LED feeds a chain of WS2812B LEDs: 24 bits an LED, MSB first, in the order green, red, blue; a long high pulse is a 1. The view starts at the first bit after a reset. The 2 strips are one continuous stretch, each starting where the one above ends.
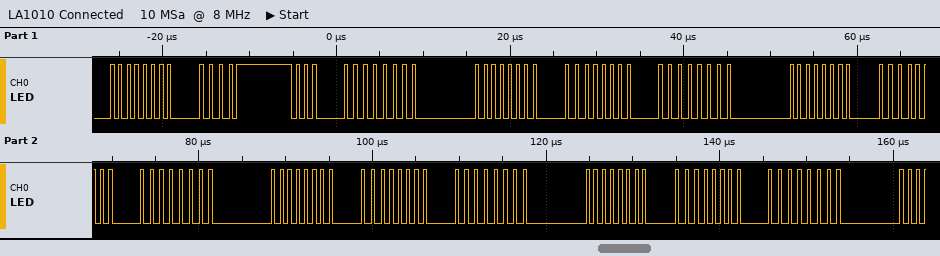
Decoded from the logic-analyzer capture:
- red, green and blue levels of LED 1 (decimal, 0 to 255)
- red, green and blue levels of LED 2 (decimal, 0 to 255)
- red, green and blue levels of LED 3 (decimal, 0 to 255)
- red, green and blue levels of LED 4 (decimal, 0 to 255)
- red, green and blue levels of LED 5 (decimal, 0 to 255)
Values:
8, 0, 0
0, 0, 0
0, 0, 0
0, 0, 0
0, 0, 0
